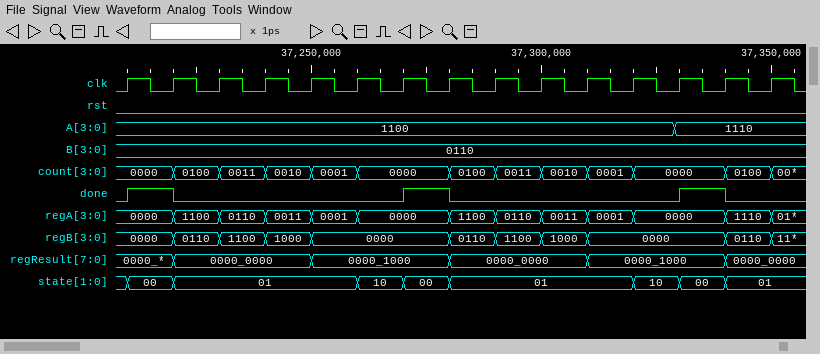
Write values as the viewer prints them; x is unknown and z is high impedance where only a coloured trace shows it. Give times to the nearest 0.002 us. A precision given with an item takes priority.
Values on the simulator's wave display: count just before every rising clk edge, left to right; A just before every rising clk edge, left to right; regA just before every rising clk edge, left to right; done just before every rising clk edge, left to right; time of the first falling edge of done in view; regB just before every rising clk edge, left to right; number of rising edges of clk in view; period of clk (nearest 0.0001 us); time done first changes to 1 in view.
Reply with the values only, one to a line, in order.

0000, 0000, 0100, 0011, 0010, 0001, 0000, 0000, 0100, 0011, 0010, 0001, 0000, 0000, 0100
1100, 1100, 1100, 1100, 1100, 1100, 1100, 1100, 1100, 1100, 1100, 1100, 1110, 1110, 1110
0000, 0000, 1100, 0110, 0011, 0001, 0000, 0000, 1100, 0110, 0011, 0001, 0000, 0000, 1110
0 1 0 0 0 0 0 1 0 0 0 0 0 1 0
37.22 us
0000, 0000, 0110, 1100, 1000, 0000, 0000, 0000, 0110, 1100, 1000, 0000, 0000, 0000, 0110
15
0.01 us
37.21 us
